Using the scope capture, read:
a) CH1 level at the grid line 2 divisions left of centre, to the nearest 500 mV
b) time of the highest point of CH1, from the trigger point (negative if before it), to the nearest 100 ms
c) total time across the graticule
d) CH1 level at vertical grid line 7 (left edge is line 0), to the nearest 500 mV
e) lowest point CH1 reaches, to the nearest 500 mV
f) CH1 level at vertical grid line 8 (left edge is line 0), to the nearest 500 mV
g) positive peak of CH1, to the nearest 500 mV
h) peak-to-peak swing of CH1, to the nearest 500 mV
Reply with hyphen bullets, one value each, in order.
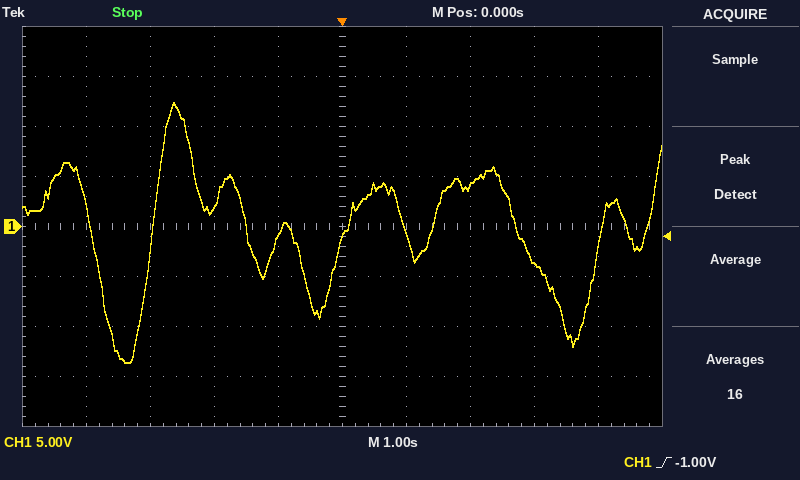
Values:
- 2.0 V
- -2.6 s
- 10 s
- 4.0 V
- -13.5 V
- -3.5 V
- 12.5 V
- 26.0 V
